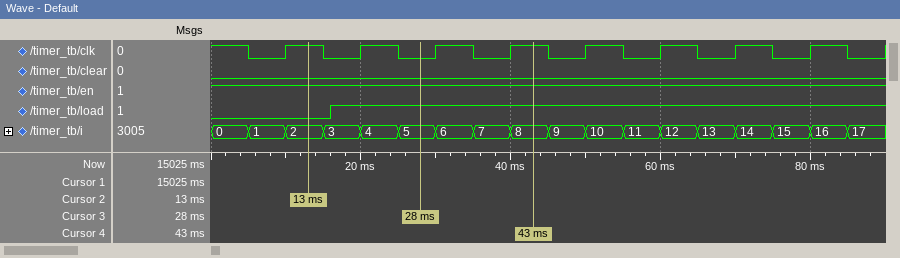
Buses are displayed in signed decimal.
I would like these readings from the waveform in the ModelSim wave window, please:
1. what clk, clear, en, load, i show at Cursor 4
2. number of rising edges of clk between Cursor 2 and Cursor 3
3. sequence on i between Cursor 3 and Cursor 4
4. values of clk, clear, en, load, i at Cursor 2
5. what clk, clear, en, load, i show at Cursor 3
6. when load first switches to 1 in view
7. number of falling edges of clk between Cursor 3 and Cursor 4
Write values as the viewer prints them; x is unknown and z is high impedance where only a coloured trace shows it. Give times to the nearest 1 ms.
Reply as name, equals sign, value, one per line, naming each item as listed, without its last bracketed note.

what clk, clear, en, load, i show at Cursor 4 = clk=1, clear=0, en=1, load=1, i=8
number of rising edges of clk between Cursor 2 and Cursor 3 = 1
sequence on i between Cursor 3 and Cursor 4 = 5, 6, 7, 8
values of clk, clear, en, load, i at Cursor 2 = clk=1, clear=0, en=1, load=0, i=2
what clk, clear, en, load, i show at Cursor 3 = clk=0, clear=0, en=1, load=1, i=5
when load first switches to 1 in view = 16 ms
number of falling edges of clk between Cursor 3 and Cursor 4 = 1
